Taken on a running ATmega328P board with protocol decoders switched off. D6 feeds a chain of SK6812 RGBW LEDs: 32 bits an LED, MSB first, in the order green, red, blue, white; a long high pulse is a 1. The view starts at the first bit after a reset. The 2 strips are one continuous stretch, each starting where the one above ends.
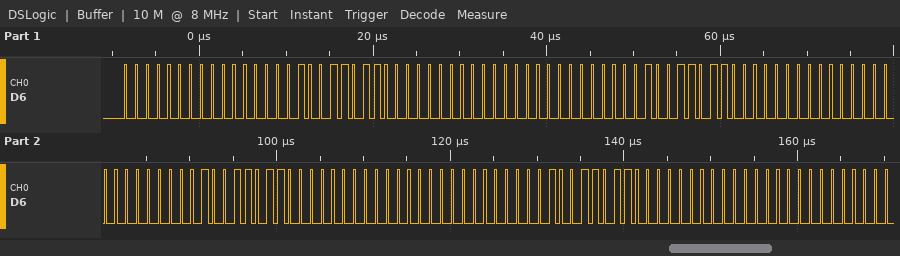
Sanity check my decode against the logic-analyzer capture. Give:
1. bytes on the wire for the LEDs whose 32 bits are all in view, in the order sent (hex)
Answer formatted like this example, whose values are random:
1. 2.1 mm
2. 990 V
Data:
1. 00 00 9B 00 00 00 9B 00 00 00 9B 00 00 00 9B 00
